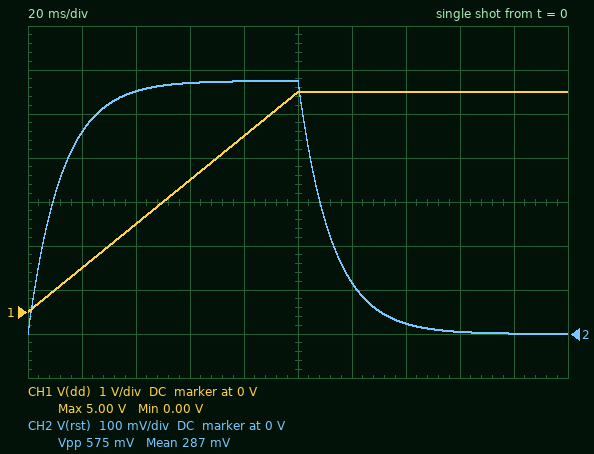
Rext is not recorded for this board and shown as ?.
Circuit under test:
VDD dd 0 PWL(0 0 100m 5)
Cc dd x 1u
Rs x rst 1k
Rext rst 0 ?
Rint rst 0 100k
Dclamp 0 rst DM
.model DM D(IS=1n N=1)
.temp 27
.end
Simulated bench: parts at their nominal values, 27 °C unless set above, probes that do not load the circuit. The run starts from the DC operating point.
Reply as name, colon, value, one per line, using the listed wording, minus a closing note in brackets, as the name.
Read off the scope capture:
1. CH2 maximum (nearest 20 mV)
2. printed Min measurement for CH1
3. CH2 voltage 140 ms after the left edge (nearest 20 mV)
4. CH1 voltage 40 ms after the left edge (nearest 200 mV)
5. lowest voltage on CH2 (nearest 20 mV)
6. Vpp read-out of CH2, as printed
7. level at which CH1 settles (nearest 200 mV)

CH2 maximum: 580 mV
printed Min measurement for CH1: 0.00 V
CH2 voltage 140 ms after the left edge: 20 mV
CH1 voltage 40 ms after the left edge: 2.0 V
lowest voltage on CH2: 0 V
Vpp read-out of CH2, as printed: 575 mV
level at which CH1 settles: 5.0 V
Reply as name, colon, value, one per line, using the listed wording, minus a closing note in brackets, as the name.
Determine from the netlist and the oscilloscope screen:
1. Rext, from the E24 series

Rext, from the E24 series: 13 kΩ
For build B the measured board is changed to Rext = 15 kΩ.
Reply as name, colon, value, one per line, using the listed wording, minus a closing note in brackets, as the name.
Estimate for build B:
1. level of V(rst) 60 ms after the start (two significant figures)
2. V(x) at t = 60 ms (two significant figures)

level of V(rst) 60 ms after the start: 640 mV
V(x) at t = 60 ms: 690 mV
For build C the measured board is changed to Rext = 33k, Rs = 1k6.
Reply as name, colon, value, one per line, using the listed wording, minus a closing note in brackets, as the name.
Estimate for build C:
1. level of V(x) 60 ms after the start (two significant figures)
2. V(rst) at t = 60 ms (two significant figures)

level of V(x) 60 ms after the start: 1.2 V
V(rst) at t = 60 ms: 1.1 V
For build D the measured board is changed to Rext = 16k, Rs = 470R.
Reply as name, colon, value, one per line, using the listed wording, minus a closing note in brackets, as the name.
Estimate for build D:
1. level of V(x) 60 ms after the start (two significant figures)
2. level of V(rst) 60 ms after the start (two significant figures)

level of V(x) 60 ms after the start: 700 mV
level of V(rst) 60 ms after the start: 680 mV
